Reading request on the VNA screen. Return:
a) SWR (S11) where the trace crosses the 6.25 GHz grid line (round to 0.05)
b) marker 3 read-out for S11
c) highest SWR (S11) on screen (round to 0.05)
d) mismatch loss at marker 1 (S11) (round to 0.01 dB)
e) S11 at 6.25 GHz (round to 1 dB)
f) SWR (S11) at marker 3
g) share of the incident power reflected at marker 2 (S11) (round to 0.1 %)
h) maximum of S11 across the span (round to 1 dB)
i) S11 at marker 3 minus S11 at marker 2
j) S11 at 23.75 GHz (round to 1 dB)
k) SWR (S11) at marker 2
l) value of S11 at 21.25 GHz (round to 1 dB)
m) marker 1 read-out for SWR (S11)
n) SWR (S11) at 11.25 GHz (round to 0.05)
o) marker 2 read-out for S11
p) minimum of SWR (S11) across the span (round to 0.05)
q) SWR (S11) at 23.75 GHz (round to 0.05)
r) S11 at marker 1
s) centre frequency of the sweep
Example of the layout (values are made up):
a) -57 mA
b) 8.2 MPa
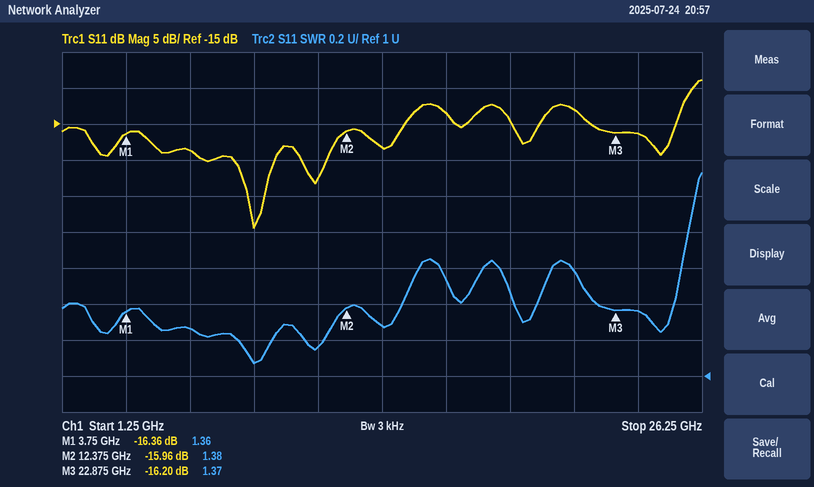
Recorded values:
a) 1.25
b) -16.20 dB
c) 2.15
d) 0.10 dB
e) -19 dB
f) 1.37
g) 2.5 %
h) -9 dB
i) -0.24 dB
j) -16 dB
k) 1.38
l) -13 dB
m) 1.36
n) 1.15
o) -15.96 dB
p) 1.05
q) 1.35
r) -16.36 dB
s) 13.75 GHz
